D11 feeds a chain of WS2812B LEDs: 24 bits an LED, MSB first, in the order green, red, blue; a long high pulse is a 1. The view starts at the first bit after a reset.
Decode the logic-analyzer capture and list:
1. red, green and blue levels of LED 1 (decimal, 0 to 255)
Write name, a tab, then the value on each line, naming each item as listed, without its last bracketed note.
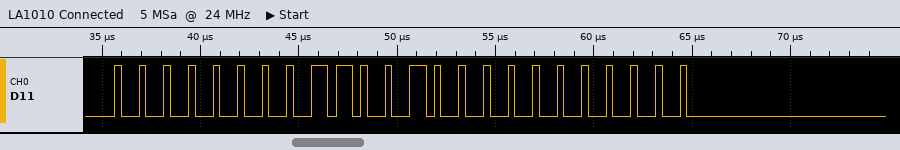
red, green and blue levels of LED 1	200, 0, 0
